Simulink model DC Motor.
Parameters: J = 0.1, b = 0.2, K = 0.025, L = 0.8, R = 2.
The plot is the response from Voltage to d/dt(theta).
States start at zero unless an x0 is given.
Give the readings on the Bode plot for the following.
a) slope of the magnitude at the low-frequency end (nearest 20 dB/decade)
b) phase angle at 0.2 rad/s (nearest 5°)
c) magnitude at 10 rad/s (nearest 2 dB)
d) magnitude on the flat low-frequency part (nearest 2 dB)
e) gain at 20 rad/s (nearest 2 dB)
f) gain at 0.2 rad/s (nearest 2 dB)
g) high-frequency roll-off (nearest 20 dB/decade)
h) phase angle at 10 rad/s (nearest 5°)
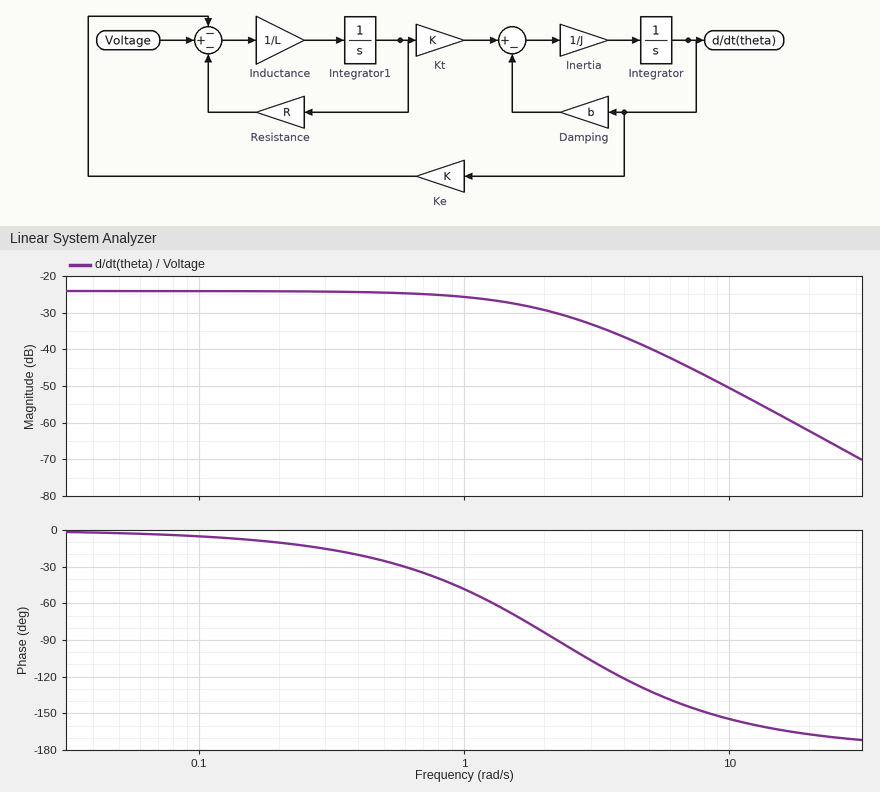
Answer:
0 dB/decade
-10°
-50 dB
-24 dB
-62 dB
-24 dB
-40 dB/decade
-155°
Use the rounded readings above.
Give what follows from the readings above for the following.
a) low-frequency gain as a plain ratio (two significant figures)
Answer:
0.063
